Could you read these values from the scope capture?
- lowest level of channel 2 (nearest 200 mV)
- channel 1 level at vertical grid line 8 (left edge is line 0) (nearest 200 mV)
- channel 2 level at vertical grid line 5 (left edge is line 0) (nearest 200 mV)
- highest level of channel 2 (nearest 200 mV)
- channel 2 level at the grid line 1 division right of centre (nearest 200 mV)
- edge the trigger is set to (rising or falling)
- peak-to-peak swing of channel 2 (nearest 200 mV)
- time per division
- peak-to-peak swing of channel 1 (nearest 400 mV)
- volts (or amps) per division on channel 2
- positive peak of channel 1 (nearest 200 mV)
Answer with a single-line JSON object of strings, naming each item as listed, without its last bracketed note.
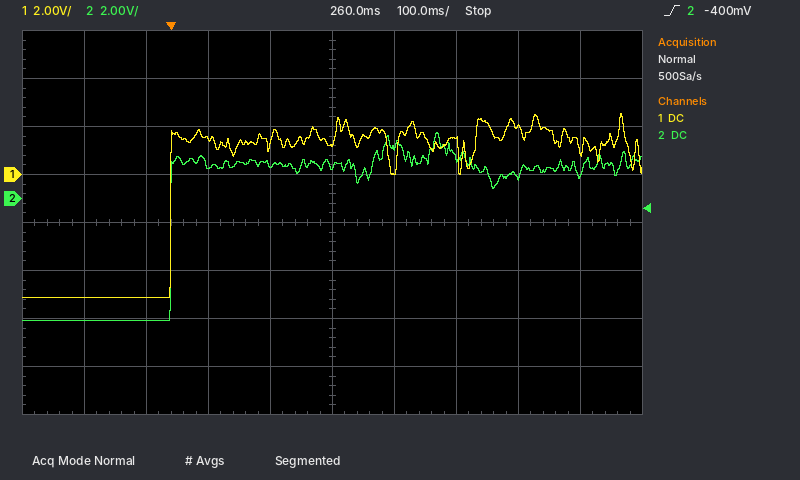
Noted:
{"lowest level of channel 2": "-5.0 V", "channel 1 level at vertical grid line 8 (left edge is line 0)": "2.0 V", "channel 2 level at vertical grid line 5 (left edge is line 0)": "1.4 V", "highest level of channel 2": "2.8 V", "channel 2 level at the grid line 1 division right of centre": "2.2 V", "edge the trigger is set to": "rising", "peak-to-peak swing of channel 2": "7.8 V", "time per division": "100 ms", "peak-to-peak swing of channel 1": "7.6 V", "volts (or amps) per division on channel 2": "2 V", "positive peak of channel 1": "2.6 V"}
